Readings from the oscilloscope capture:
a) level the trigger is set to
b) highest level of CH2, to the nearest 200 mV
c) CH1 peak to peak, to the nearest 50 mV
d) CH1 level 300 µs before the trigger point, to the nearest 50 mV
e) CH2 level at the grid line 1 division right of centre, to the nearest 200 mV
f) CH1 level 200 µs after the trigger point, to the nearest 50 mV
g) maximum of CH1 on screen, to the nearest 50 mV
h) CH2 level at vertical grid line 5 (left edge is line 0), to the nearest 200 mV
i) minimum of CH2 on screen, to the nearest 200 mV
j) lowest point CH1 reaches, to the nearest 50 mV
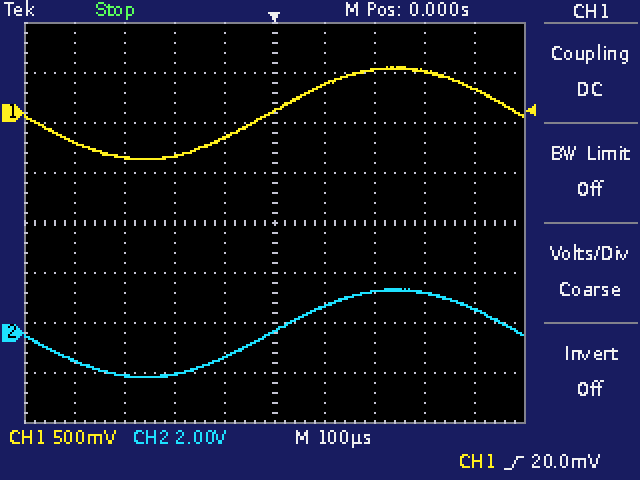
20.0 mV
1.8 V
900 mV
-450 mV
1.0 V
450 mV
450 mV
0.0 V
-1.8 V
-450 mV
